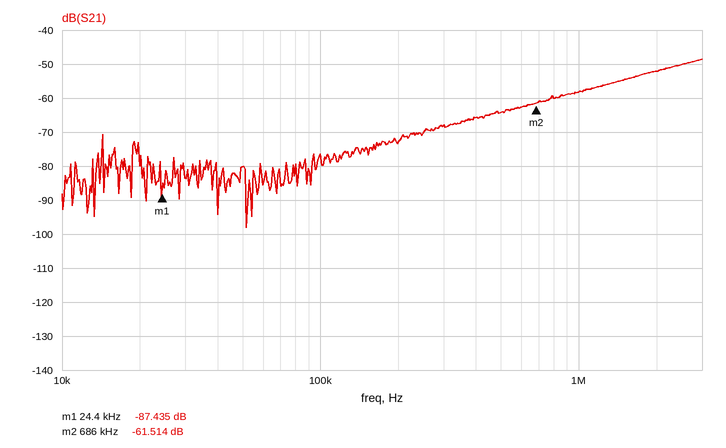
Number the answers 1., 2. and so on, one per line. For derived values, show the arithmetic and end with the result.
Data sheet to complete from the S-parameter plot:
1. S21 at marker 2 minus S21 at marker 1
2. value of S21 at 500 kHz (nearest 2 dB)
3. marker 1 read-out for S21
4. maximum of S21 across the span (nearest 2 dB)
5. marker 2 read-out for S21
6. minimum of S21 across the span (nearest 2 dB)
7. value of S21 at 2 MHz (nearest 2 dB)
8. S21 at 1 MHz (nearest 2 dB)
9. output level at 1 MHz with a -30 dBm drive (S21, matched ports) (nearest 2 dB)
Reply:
1. -61.514 − (-87.435) = 25.921 dB
2. -64 dB
3. -87.435 dB
4. -48 dB
5. -61.514 dB
6. -98 dB
7. -52 dB
8. -58 dB
9. -30 dBm + (-58 dB) = -88 dBm
